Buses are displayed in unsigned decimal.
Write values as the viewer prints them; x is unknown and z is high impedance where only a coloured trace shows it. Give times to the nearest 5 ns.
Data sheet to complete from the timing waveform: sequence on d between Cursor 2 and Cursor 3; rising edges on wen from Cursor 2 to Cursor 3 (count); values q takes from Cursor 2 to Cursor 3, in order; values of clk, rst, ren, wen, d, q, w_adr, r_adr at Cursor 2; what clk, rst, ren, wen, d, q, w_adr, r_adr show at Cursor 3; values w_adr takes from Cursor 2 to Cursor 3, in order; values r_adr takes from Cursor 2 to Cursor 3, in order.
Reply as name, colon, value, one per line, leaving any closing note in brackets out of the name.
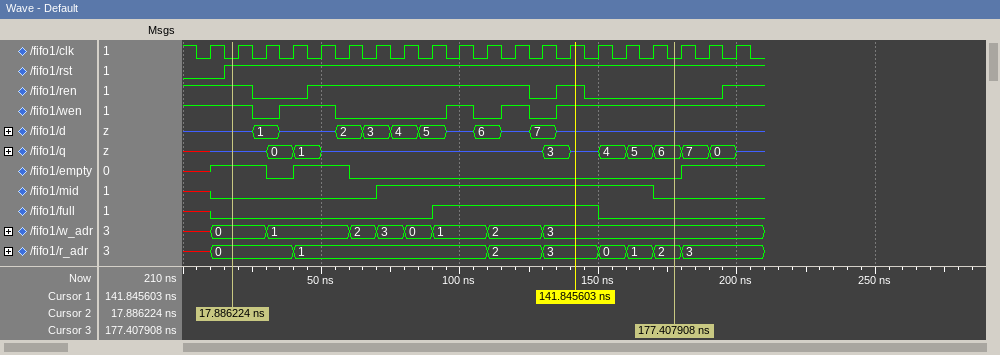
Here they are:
sequence on d between Cursor 2 and Cursor 3: z, 1, z, 2, 3, 4, 5, z, 6, z, 7, z
rising edges on wen from Cursor 2 to Cursor 3: 4
values q takes from Cursor 2 to Cursor 3, in order: z, 0, 1, z, 3, z, 4, 5, 6
values of clk, rst, ren, wen, d, q, w_adr, r_adr at Cursor 2: clk=0, rst=1, ren=1, wen=1, d=z, q=z, w_adr=0, r_adr=0
what clk, rst, ren, wen, d, q, w_adr, r_adr show at Cursor 3: clk=0, rst=1, ren=0, wen=1, d=z, q=6, w_adr=3, r_adr=2
values w_adr takes from Cursor 2 to Cursor 3, in order: 0, 1, 2, 3, 0, 1, 2, 3
values r_adr takes from Cursor 2 to Cursor 3, in order: 0, 1, 2, 3, 0, 1, 2
